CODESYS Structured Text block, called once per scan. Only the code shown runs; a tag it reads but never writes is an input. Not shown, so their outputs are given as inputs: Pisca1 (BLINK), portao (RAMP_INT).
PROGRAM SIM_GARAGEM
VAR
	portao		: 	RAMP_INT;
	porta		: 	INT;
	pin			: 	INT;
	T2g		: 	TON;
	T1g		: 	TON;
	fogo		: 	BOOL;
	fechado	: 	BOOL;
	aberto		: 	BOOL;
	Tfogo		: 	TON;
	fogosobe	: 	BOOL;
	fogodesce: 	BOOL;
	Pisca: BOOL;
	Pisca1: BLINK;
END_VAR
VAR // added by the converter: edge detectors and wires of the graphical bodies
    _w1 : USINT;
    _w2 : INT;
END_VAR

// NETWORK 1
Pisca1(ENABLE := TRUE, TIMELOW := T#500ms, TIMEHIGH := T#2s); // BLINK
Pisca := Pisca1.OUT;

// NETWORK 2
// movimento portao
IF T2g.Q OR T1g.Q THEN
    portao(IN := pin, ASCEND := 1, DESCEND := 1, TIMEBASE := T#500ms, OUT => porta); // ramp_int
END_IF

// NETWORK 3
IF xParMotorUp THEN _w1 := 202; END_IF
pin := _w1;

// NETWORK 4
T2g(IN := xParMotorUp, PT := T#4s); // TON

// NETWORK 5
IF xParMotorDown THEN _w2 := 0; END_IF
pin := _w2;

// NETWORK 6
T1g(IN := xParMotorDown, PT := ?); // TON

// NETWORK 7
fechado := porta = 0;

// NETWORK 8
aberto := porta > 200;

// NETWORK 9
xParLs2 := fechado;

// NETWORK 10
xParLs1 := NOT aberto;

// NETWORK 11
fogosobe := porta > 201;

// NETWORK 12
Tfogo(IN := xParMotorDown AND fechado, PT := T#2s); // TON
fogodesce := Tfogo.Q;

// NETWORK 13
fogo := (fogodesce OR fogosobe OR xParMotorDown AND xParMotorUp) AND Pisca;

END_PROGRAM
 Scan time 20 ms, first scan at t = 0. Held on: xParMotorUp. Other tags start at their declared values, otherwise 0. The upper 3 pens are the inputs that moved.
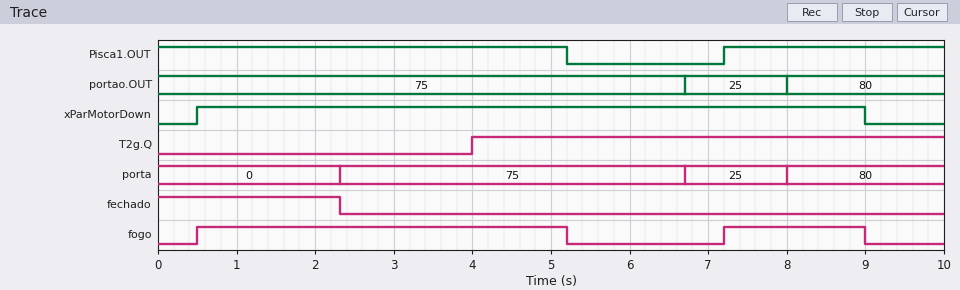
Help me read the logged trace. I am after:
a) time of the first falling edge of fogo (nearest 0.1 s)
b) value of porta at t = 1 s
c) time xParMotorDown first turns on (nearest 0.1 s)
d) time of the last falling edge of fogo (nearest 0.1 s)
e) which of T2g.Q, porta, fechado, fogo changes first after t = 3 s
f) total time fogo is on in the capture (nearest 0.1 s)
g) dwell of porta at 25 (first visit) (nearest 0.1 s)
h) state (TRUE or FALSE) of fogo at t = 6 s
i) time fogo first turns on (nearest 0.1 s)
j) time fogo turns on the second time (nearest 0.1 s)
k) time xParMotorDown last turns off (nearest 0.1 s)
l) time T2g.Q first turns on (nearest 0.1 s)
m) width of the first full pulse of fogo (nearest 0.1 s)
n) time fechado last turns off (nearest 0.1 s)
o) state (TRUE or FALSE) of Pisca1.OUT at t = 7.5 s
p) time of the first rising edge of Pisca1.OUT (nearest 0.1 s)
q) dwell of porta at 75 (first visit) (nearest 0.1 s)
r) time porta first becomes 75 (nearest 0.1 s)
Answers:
5.2 s
0
0.5 s
9.0 s
T2g.Q
6.5 s
1.3 s
FALSE
0.5 s
7.2 s
9.0 s
4.0 s
4.7 s
2.3 s
TRUE
7.2 s
4.4 s
2.3 s
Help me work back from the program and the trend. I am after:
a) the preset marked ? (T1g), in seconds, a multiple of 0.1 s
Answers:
1.8 s
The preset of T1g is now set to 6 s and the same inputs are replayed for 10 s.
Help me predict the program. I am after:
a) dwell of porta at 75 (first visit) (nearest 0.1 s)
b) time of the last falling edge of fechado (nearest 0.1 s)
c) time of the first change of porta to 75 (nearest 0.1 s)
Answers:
2.7 s
4.0 s
4.0 s
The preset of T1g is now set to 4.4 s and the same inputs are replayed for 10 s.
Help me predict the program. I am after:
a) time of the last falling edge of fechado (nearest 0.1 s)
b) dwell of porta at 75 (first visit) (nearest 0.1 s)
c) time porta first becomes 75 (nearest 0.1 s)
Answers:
4.0 s
2.7 s
4.0 s
